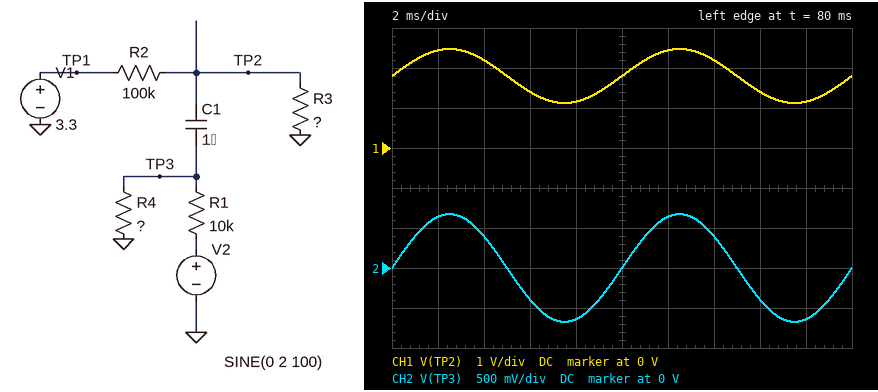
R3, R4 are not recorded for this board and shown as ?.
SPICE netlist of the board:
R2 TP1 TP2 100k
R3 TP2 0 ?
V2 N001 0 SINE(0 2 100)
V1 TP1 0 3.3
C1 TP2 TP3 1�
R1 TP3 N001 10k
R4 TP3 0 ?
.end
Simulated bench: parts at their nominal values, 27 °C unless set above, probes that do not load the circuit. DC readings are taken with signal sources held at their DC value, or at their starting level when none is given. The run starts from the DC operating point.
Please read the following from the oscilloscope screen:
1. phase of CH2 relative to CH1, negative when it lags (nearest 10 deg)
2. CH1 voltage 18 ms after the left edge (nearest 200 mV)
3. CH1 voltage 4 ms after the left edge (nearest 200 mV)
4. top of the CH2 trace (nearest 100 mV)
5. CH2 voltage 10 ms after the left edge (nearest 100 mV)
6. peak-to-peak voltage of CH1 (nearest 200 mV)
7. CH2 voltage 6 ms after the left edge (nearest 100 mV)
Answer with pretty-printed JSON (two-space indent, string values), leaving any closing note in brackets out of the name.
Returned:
{
  "phase of CH2 relative to CH1, negative when it lags": "0 deg",
  "CH1 voltage 18 ms after the left edge": "1.2 V",
  "CH1 voltage 4 ms after the left edge": "2.2 V",
  "top of the CH2 trace": "700 mV",
  "CH2 voltage 10 ms after the left edge": "0 V",
  "peak-to-peak voltage of CH1": "1.4 V",
  "CH2 voltage 6 ms after the left edge": "-400 mV"
}
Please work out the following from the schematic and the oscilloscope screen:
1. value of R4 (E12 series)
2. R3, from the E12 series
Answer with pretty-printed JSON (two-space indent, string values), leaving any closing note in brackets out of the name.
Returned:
{
  "value of R4": "5.6 kΩ",
  "R3, from the E12 series": "120 kΩ"
}
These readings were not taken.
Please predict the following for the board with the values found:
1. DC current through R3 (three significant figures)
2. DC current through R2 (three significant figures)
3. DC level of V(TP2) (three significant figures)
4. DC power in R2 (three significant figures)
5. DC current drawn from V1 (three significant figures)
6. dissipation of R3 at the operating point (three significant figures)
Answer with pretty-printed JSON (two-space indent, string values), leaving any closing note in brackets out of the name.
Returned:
{
  "DC current through R3": "15.0 µA",
  "DC current through R2": "15.0 µA",
  "DC level of V(TP2)": "1.80 V",
  "DC power in R2": "22.5 µW",
  "DC current drawn from V1": "15.0 µA",
  "dissipation of R3 at the operating point": "27.0 µW"
}
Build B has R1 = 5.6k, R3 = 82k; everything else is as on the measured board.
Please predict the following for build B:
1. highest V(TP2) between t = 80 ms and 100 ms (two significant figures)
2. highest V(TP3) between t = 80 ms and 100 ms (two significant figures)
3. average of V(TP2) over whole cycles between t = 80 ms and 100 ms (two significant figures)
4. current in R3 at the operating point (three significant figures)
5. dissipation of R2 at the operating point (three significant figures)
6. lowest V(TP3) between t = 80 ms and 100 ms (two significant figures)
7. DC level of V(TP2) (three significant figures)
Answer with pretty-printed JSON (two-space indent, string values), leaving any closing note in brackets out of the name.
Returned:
{
  "highest V(TP2) between t = 80 ms and 100 ms": "2.4 V",
  "highest V(TP3) between t = 80 ms and 100 ms": "940 mV",
  "average of V(TP2) over whole cycles between t = 80 ms and 100 ms": "1.5 V",
  "current in R3 at the operating point": "18.1 µA",
  "dissipation of R2 at the operating point": "32.9 µW",
  "lowest V(TP3) between t = 80 ms and 100 ms": "-940 mV",
  "DC level of V(TP2)": "1.49 V"
}
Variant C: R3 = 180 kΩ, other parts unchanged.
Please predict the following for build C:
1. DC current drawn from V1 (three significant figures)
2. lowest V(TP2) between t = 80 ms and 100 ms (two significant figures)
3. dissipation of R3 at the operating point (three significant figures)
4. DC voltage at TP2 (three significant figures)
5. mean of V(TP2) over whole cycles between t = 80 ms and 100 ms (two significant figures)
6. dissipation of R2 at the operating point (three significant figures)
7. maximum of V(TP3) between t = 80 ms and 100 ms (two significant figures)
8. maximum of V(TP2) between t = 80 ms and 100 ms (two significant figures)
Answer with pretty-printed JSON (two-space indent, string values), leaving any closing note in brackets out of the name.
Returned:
{
  "DC current drawn from V1": "11.8 µA",
  "lowest V(TP2) between t = 80 ms and 100 ms": "1.4 V",
  "dissipation of R3 at the operating point": "25.0 µW",
  "DC voltage at TP2": "2.12 V",
  "mean of V(TP2) over whole cycles between t = 80 ms and 100 ms": "2.1 V",
  "dissipation of R2 at the operating point": "13.9 µW",
  "maximum of V(TP3) between t = 80 ms and 100 ms": "680 mV",
  "maximum of V(TP2) between t = 80 ms and 100 ms": "2.8 V"
}
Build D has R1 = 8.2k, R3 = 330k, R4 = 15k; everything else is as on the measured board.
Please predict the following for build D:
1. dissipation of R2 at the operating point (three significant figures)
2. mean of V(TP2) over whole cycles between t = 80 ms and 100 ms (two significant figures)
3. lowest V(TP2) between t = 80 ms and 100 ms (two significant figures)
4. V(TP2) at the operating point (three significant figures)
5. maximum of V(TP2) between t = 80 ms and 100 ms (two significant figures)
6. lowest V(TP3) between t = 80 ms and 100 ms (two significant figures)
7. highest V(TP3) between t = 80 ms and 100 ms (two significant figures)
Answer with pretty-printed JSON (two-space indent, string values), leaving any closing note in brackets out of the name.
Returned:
{
  "dissipation of R2 at the operating point": "5.89 µW",
  "mean of V(TP2) over whole cycles between t = 80 ms and 100 ms": "2.5 V",
  "lowest V(TP2) between t = 80 ms and 100 ms": "1.3 V",
  "V(TP2) at the operating point": "2.53 V",
  "maximum of V(TP2) between t = 80 ms and 100 ms": "3.7 V",
  "lowest V(TP3) between t = 80 ms and 100 ms": "-1.2 V",
  "highest V(TP3) between t = 80 ms and 100 ms": "1.2 V"
}
